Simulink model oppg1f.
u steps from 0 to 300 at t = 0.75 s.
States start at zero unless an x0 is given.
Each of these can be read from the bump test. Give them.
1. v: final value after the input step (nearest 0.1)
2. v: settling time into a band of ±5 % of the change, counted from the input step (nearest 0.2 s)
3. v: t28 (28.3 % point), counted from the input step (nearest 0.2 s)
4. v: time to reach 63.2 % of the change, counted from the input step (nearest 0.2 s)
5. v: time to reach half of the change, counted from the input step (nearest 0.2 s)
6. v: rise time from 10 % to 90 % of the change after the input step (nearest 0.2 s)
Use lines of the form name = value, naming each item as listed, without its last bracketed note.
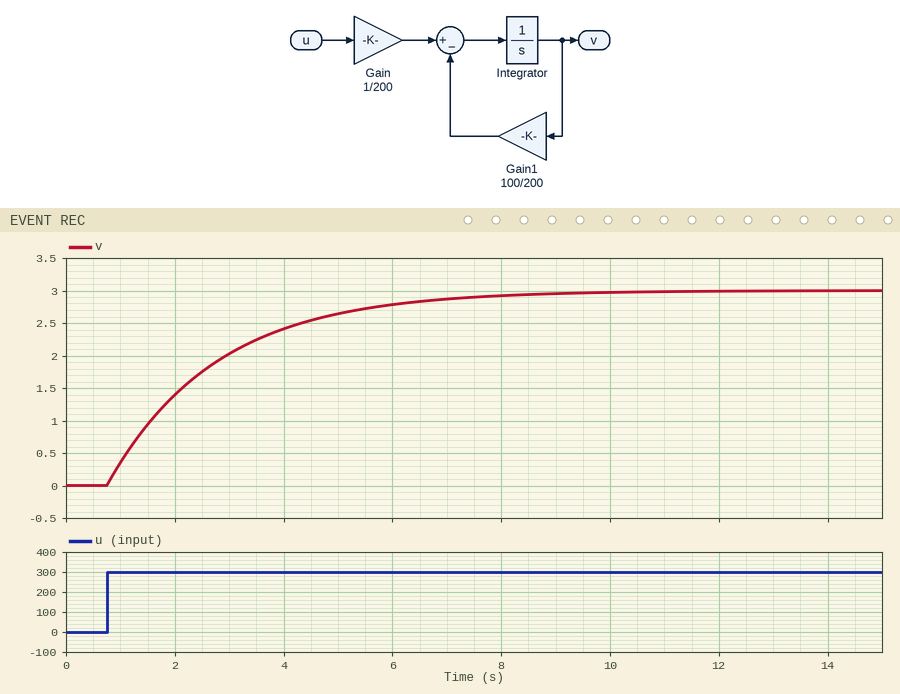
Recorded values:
v: final value after the input step = 3.0
v: settling time into a band of ±5 % of the change, counted from the input step = 6.0 s
v: t28 (28.3 % point), counted from the input step = 0.6 s
v: time to reach 63.2 % of the change, counted from the input step = 2.0 s
v: time to reach half of the change, counted from the input step = 1.4 s
v: rise time from 10 % to 90 % of the change after the input step = 4.4 s
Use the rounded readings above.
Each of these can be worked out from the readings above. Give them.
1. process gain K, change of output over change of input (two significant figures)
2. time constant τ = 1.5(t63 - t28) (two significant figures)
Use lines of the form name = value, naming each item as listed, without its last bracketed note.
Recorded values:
process gain K, change of output over change of input = 0.010
time constant τ = 1.5(t63 - t28) = 2.1 s
